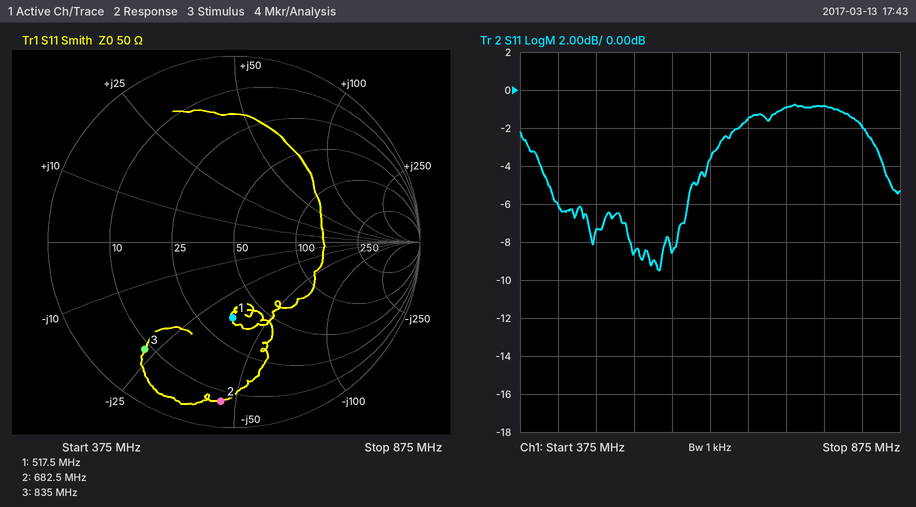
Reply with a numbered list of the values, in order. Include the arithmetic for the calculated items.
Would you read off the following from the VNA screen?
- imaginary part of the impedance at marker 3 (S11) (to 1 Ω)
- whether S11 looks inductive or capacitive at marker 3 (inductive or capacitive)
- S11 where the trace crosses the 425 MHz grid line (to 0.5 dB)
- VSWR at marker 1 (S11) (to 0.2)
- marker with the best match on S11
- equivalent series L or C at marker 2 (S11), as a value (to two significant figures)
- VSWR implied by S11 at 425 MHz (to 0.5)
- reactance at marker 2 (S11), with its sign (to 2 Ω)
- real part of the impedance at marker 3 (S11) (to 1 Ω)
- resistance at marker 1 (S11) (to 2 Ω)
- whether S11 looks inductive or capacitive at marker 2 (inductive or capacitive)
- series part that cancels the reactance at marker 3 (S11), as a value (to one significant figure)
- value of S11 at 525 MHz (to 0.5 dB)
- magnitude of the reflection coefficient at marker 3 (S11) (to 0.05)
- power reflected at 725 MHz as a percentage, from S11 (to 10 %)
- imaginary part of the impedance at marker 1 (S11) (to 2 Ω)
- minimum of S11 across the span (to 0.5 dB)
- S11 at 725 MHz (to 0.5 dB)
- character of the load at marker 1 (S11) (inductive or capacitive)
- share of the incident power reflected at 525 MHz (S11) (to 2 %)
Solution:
1. -23 Ω
2. capacitive
3. -6.0 dB
4. 2.4
5. marker 1
6. C = 1/(2π × 682.5 MHz × 46 Ω) ≈ 5.1 pF
7. |Γ| = 10^(-6/20) = 0.5012; VSWR = (1 + 0.5012)/(1 − 0.5012) ≈ 3.0
8. -46 Ω
9. 9 Ω
10. 36 Ω
11. capacitive
12. L = 23 Ω/(2π × 835 MHz) ≈ 4 nH
13. -8.5 dB
14. 0.75
15. 10^(-1/10) ≈ 79.4 %, so 80 % to the nearest 10 %
16. -34 Ω
17. -9.5 dB
18. -1.0 dB
19. capacitive
20. 10^(-8.5/10) ≈ 14 %
